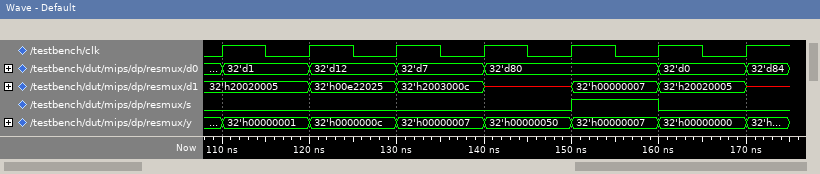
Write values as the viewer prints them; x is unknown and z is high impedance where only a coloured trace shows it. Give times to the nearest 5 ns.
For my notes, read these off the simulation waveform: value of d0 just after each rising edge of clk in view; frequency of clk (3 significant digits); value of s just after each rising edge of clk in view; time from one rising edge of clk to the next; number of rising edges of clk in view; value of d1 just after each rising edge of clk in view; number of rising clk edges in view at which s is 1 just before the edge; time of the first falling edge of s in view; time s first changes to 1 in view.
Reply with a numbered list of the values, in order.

1. 32'd1, 32'd12, 32'd7, 32'd80, 32'd80, 32'd0, 32'd84
2. 100 MHz
3. 0 0 0 0 1 0 0
4. 10 ns
5. 7
6. 32'h20020005, 32'h00e22025, 32'h2003000c, x, 32'h00000007, 32'h20020005, x
7. 1
8. 160 ns
9. 150 ns
